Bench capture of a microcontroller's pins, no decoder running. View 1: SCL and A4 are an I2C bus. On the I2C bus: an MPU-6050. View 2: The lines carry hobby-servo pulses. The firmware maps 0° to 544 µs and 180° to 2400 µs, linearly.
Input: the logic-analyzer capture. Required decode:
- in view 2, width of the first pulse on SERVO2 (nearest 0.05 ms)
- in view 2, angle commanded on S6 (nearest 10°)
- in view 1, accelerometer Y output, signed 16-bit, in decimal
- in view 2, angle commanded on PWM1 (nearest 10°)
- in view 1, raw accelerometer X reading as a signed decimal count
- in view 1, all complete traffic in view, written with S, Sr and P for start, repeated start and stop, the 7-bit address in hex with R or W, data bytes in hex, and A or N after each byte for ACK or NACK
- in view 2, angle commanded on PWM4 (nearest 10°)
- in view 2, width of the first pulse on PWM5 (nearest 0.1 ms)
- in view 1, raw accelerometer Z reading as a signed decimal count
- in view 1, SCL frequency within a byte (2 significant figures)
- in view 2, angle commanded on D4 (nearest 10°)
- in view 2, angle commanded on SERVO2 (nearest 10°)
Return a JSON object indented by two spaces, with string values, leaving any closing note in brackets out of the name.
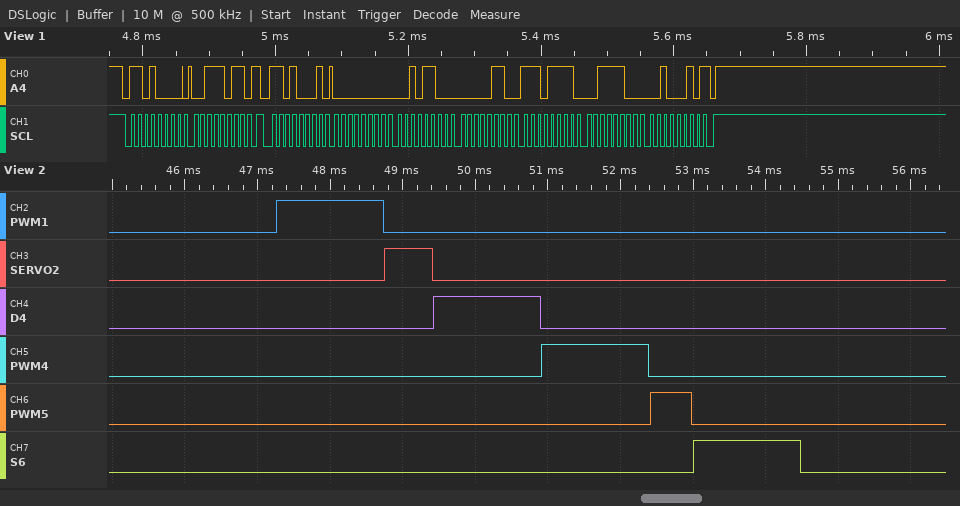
{
  "in view 2, width of the first pulse on SERVO2": "0.65 ms",
  "in view 2, angle commanded on S6": "90°",
  "in view 1, accelerometer Y output, signed 16-bit, in decimal": "1775",
  "in view 2, angle commanded on PWM1": "90°",
  "in view 1, raw accelerometer X reading as a signed decimal count": "44",
  "in view 1, all complete traffic in view, written with S, Sr and P for start, repeated start and stop, the 7-bit address in hex with R or W, data bytes in hex, and A or N after each byte for ACK or NACK": "S 68W A 3B A Sr 68R A 00 A 2C A 06 A EF A 3C A 22 N P",
  "in view 2, angle commanded on PWM4": "90°",
  "in view 2, width of the first pulse on PWM5": "0.6 ms",
  "in view 1, raw accelerometer Z reading as a signed decimal count": "15394",
  "in view 1, SCL frequency within a byte": "100 kHz",
  "in view 2, angle commanded on D4": "90°",
  "in view 2, angle commanded on SERVO2": "10°"
}
